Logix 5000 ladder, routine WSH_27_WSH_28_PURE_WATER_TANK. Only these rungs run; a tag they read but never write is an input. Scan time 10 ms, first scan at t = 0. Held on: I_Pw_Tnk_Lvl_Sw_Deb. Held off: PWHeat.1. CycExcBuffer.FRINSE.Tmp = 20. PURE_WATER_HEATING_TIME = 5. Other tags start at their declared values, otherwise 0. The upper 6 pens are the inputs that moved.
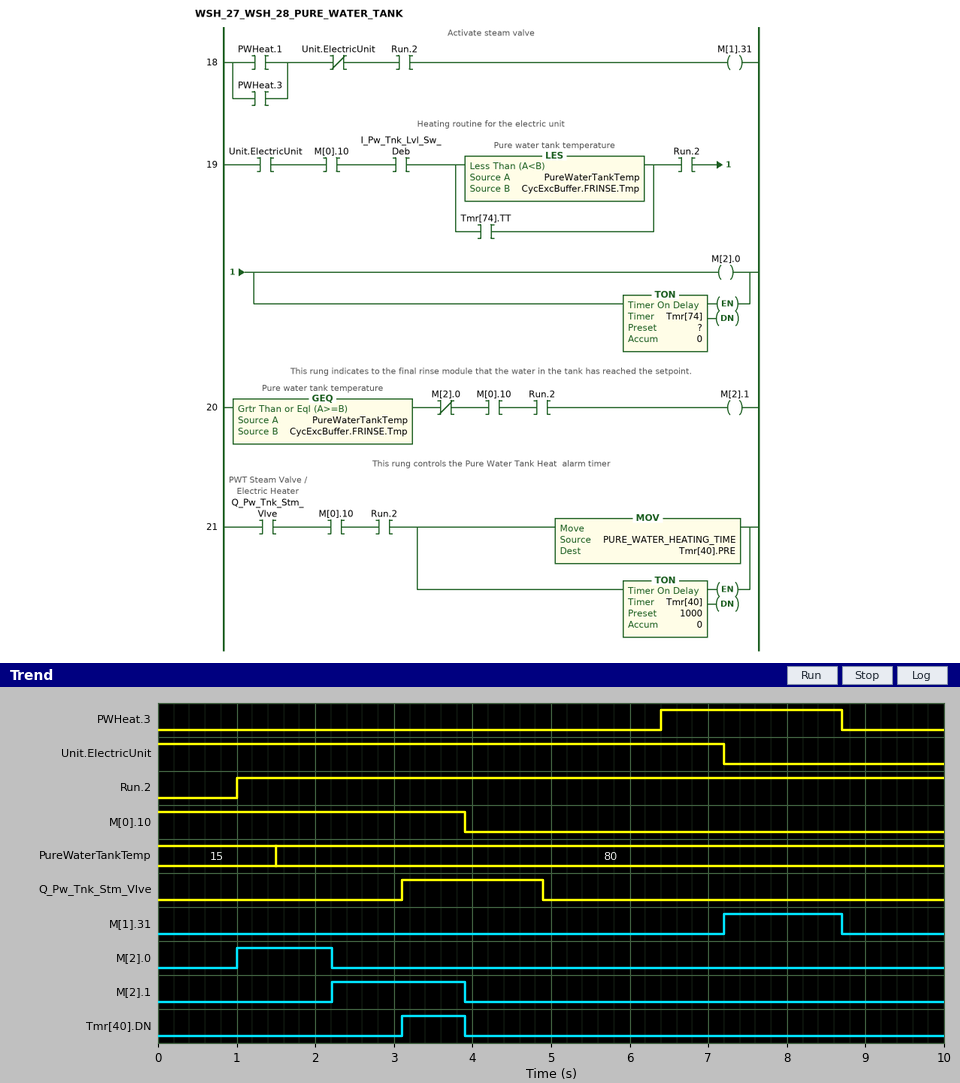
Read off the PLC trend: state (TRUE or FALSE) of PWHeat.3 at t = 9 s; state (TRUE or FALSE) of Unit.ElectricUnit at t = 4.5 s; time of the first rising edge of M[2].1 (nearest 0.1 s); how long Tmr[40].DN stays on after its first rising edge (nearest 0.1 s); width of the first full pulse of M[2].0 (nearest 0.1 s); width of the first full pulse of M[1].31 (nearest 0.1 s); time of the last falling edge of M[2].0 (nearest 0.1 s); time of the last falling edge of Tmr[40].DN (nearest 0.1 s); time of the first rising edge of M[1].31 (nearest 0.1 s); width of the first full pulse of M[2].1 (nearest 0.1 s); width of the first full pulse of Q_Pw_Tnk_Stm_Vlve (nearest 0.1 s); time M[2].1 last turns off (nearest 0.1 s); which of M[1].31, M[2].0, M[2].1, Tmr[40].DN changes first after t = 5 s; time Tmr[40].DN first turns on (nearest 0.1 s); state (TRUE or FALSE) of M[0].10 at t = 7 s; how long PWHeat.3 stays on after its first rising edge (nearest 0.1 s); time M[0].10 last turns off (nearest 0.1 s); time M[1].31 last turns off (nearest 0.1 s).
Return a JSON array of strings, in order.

["FALSE", "TRUE", "2.2 s", "0.8 s", "1.2 s", "1.5 s", "2.2 s", "3.9 s", "7.2 s", "1.7 s", "1.8 s", "3.9 s", "M[1].31", "3.1 s", "FALSE", "2.3 s", "3.9 s", "8.7 s"]
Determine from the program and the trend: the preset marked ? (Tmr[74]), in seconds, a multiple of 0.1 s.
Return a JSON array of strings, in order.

["1.2 s"]
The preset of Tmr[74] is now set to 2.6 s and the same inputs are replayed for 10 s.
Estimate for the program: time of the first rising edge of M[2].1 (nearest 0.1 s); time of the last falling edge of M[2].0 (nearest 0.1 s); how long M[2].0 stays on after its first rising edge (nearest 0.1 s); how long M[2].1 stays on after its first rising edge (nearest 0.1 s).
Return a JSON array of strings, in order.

["3.6 s", "3.6 s", "2.6 s", "0.3 s"]
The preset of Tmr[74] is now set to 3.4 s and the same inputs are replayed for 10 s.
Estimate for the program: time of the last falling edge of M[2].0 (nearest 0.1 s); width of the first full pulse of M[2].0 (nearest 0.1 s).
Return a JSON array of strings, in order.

["3.9 s", "2.9 s"]
